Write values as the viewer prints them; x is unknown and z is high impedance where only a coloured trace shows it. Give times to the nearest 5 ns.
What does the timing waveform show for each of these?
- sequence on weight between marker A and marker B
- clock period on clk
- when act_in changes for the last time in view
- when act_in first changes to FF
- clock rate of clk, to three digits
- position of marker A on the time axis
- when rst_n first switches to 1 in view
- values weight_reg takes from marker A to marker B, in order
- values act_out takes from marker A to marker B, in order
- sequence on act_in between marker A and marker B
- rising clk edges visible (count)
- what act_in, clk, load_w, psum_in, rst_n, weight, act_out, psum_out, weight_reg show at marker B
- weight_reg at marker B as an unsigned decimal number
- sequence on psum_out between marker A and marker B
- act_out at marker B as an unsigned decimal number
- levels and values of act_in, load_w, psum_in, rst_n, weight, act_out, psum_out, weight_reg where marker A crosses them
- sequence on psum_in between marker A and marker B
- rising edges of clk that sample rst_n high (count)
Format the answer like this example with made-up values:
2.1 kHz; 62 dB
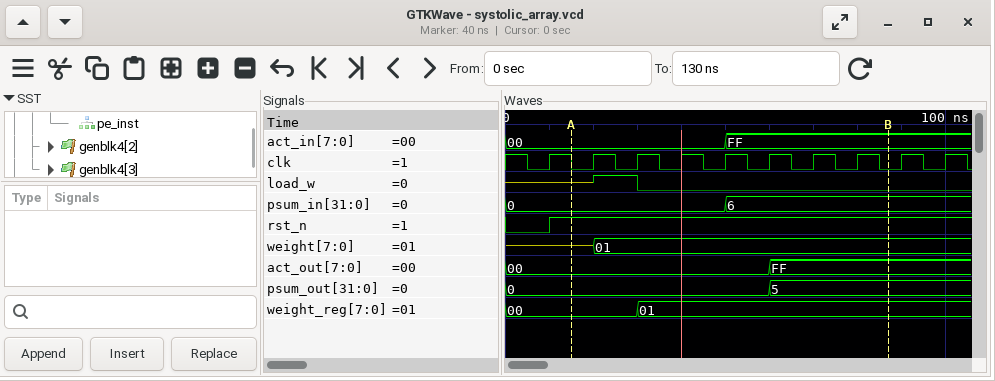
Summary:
z, 01; 10 ns; 50 ns; 50 ns; 100 MHz; 15 ns; 10 ns; 00, 01; 00, FF; 00, FF; 10; act_in=FF, clk=0, load_w=0, psum_in=6, rst_n=1, weight=01, act_out=FF, psum_out=5, weight_reg=01; 1; 0, 5; 255; act_in=00, load_w=z, psum_in=0, rst_n=1, weight=z, act_out=00, psum_out=0, weight_reg=00; 0, 6; 9
